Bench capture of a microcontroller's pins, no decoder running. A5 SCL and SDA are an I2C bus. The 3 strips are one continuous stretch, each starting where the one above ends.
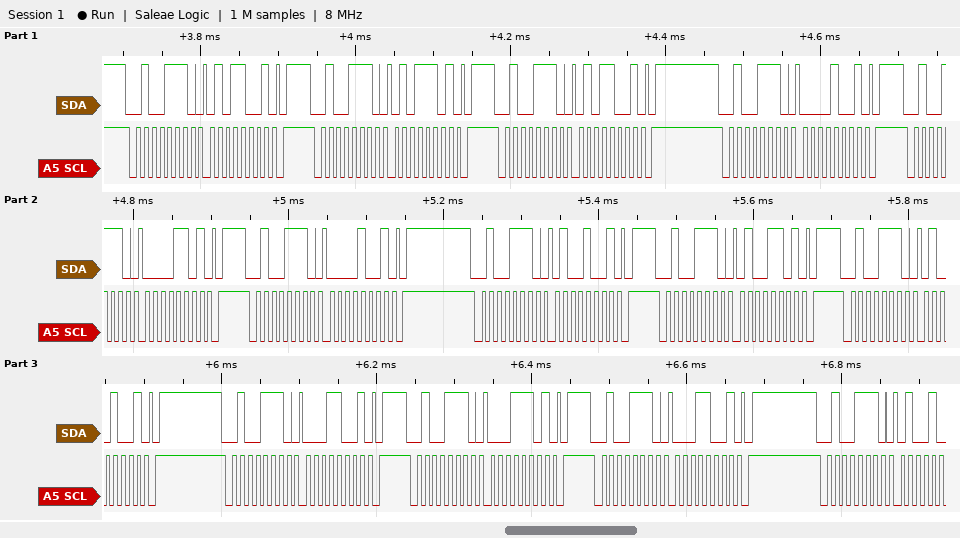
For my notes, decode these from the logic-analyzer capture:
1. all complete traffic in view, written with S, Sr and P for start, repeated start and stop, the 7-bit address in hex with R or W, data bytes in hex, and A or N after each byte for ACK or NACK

S 27W A 59 A P S 27W A 5D A P S 27W A 59 A P S 27W A 09 A P S 27W A 0D A P S 27W A 09 A P S 27W A 49 A P S 27W A 4D A P S 27W A 49 A P S 27W A 19 A P S 27W A 1D A P S 27W A 19 A P S 27W A
